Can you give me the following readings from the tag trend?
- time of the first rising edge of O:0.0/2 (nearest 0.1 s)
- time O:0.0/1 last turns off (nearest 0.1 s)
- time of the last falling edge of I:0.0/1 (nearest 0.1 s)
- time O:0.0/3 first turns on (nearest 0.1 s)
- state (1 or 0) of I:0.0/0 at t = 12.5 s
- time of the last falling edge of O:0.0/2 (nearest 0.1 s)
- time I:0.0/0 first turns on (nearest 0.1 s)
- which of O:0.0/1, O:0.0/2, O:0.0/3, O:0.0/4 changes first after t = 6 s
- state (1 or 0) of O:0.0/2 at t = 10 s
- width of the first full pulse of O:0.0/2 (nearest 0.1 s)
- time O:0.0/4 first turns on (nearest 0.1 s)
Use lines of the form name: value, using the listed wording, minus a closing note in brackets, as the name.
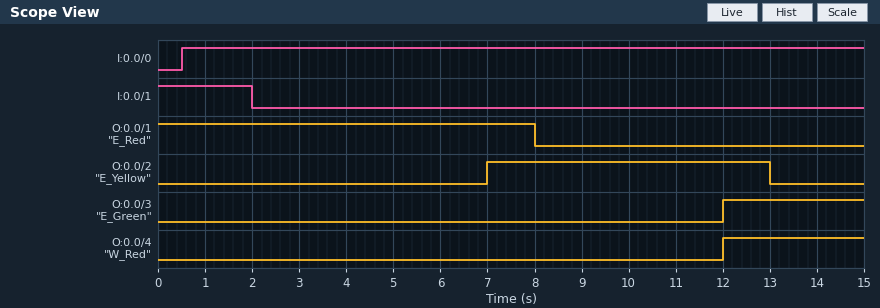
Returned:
time of the first rising edge of O:0.0/2: 7.0 s
time O:0.0/1 last turns off: 8.0 s
time of the last falling edge of I:0.0/1: 2.0 s
time O:0.0/3 first turns on: 12.0 s
state (1 or 0) of I:0.0/0 at t = 12.5 s: 1
time of the last falling edge of O:0.0/2: 13.0 s
time I:0.0/0 first turns on: 0.5 s
which of O:0.0/1, O:0.0/2, O:0.0/3, O:0.0/4 changes first after t = 6 s: O:0.0/2
state (1 or 0) of O:0.0/2 at t = 10 s: 1
width of the first full pulse of O:0.0/2: 6.0 s
time O:0.0/4 first turns on: 12.0 s
